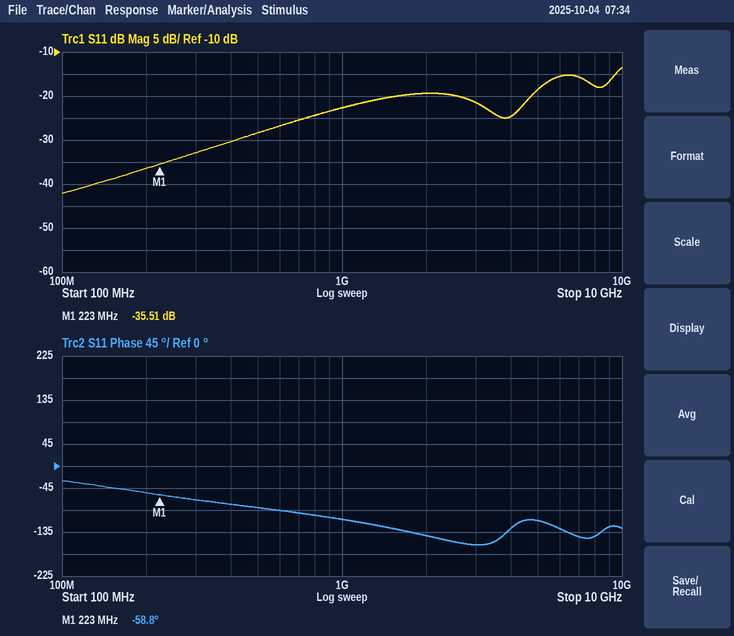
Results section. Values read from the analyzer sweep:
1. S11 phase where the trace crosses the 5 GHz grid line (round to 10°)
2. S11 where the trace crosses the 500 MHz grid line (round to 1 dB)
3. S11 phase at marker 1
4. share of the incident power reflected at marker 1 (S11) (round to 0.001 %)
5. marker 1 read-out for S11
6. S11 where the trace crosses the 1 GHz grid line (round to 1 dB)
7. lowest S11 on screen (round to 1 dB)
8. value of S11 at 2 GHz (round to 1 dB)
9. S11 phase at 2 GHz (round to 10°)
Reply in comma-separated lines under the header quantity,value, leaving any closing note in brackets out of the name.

quantity,value
S11 phase where the trace crosses the 5 GHz grid line,-110°
S11 where the trace crosses the 500 MHz grid line,-28 dB
S11 phase at marker 1,-58.8°
share of the incident power reflected at marker 1 (S11),0.028 %
marker 1 read-out for S11,-35.51 dB
S11 where the trace crosses the 1 GHz grid line,-23 dB
lowest S11 on screen,-42 dB
value of S11 at 2 GHz,-19 dB
S11 phase at 2 GHz,-140°
